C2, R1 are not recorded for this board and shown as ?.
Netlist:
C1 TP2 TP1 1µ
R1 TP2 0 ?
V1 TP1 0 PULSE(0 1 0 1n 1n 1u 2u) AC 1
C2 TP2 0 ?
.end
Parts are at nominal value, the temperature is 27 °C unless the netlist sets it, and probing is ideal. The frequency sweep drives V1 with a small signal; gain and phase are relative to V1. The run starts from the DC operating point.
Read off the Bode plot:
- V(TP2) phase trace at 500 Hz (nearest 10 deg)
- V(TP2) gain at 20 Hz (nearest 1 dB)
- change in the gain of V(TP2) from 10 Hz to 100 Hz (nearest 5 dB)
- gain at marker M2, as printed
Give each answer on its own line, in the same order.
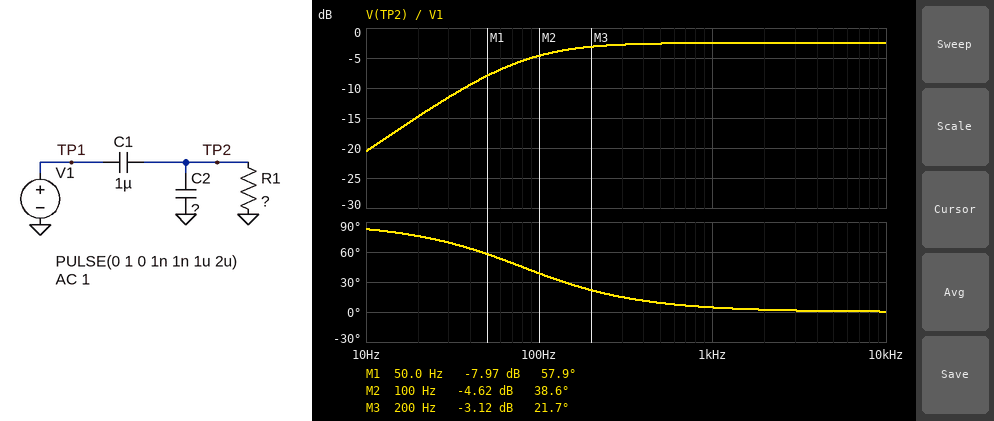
10 deg
-15 dB
15 dB
-4.62 dB
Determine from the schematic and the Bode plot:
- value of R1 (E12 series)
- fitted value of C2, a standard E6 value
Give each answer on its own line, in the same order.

1.5 kΩ
330 nF
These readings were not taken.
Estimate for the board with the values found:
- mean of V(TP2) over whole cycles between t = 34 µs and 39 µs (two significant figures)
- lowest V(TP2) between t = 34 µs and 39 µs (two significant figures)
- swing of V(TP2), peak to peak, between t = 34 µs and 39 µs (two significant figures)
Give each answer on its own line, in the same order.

370 mV
-7.1 mV
750 mV
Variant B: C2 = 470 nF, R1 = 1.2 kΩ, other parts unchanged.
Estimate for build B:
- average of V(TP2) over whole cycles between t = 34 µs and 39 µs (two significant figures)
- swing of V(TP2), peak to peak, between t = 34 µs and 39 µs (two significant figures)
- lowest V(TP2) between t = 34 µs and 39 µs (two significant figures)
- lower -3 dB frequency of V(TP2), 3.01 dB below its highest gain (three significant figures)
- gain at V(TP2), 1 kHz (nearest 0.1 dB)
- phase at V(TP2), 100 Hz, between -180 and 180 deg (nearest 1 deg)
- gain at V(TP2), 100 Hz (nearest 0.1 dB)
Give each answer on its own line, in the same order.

330 mV
680 mV
-7.3 mV
90.2 Hz
-3.4 dB
42 deg
-5.9 dB
